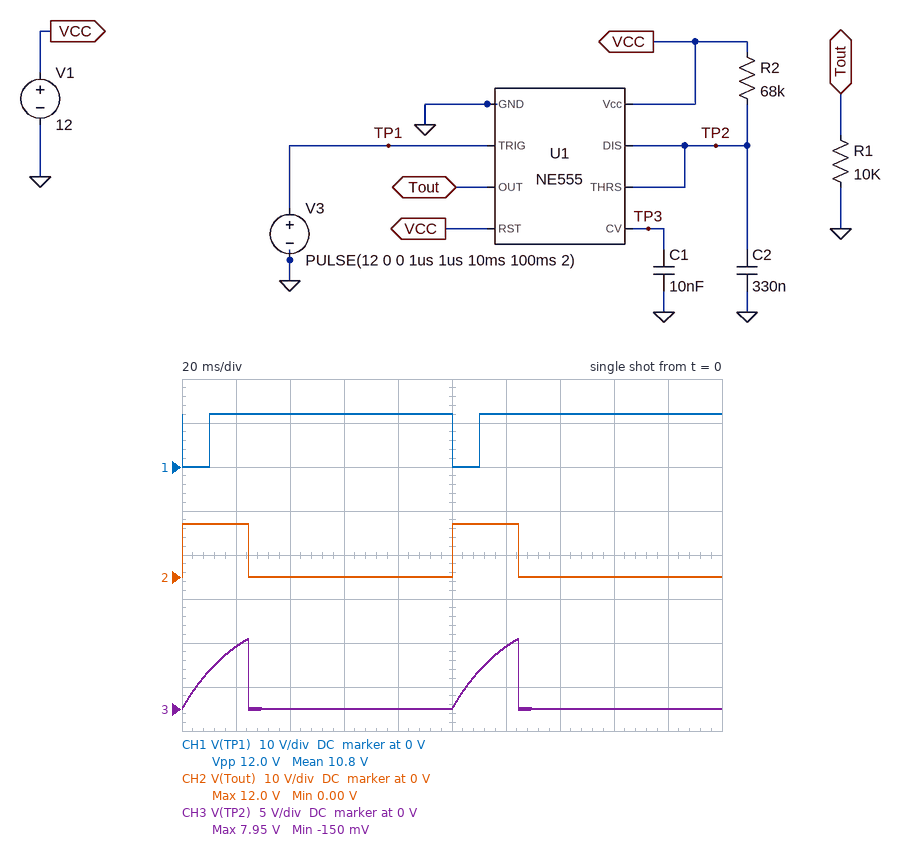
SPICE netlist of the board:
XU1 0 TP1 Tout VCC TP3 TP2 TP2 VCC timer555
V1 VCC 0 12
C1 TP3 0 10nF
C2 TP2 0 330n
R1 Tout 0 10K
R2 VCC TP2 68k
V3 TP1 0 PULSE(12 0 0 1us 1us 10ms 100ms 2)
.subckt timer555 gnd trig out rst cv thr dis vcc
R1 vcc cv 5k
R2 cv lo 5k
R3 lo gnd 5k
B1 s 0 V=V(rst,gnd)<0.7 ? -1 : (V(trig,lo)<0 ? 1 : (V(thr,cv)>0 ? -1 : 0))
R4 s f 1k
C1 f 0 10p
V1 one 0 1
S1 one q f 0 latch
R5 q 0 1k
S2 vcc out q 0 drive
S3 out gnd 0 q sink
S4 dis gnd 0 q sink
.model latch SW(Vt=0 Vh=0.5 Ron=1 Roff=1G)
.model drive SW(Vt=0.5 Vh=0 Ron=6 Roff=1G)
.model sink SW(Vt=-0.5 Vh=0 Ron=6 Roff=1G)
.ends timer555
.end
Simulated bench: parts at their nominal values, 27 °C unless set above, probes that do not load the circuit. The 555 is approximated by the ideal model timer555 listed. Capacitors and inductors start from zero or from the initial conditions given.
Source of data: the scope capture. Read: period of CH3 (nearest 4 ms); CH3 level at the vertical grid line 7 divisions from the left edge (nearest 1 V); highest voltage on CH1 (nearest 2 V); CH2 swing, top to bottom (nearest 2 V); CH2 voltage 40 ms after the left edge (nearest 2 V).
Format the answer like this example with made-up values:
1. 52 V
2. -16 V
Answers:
1. 100 ms
2. 0 V
3. 12 V
4. 12 V
5. 0 V
